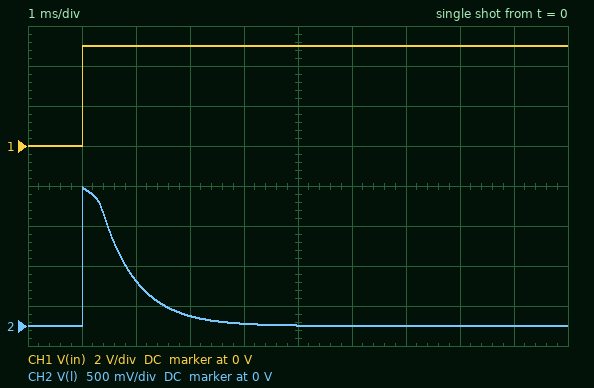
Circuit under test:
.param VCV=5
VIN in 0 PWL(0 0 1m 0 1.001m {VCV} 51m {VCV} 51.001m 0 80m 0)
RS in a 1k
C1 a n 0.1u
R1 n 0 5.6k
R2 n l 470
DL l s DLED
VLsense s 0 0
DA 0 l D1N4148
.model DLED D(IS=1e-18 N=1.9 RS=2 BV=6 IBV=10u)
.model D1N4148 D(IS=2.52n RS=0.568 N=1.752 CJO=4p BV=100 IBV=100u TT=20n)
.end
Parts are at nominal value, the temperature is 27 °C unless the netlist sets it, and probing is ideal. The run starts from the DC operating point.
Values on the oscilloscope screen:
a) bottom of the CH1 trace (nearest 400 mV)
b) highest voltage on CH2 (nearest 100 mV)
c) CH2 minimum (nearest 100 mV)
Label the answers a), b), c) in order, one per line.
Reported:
a) 0 V
b) 1.7 V
c) 0 V
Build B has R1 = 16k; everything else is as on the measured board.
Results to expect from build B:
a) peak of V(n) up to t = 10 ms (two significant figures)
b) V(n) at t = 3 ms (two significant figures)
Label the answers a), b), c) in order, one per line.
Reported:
a) 2.7 V
b) 640 mV
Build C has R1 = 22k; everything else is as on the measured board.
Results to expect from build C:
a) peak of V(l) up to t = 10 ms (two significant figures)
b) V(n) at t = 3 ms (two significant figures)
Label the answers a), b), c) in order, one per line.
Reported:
a) 1.7 V
b) 820 mV
